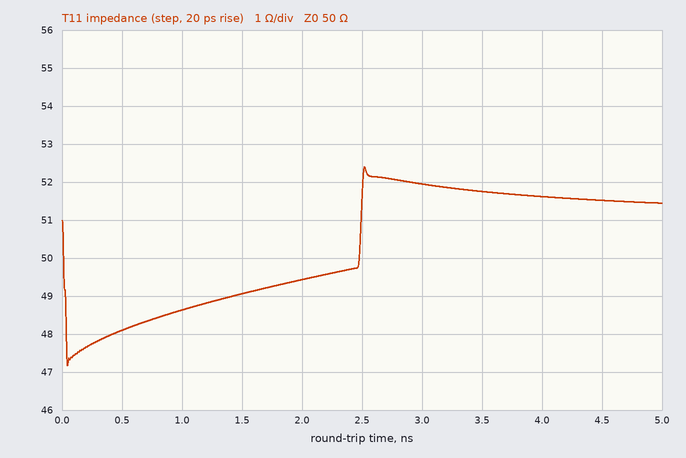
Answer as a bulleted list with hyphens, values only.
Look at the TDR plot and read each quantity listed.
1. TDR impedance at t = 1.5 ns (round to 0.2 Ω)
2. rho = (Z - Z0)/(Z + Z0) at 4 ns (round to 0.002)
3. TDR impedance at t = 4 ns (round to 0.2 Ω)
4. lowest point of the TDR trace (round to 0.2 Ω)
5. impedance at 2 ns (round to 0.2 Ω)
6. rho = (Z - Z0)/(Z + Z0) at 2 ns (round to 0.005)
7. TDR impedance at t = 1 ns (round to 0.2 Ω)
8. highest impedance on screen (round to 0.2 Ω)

- 49.0 Ω
- +0.016
- 51.6 Ω
- 47.2 Ω
- 49.4 Ω
- -0.005
- 48.6 Ω
- 52.4 Ω
